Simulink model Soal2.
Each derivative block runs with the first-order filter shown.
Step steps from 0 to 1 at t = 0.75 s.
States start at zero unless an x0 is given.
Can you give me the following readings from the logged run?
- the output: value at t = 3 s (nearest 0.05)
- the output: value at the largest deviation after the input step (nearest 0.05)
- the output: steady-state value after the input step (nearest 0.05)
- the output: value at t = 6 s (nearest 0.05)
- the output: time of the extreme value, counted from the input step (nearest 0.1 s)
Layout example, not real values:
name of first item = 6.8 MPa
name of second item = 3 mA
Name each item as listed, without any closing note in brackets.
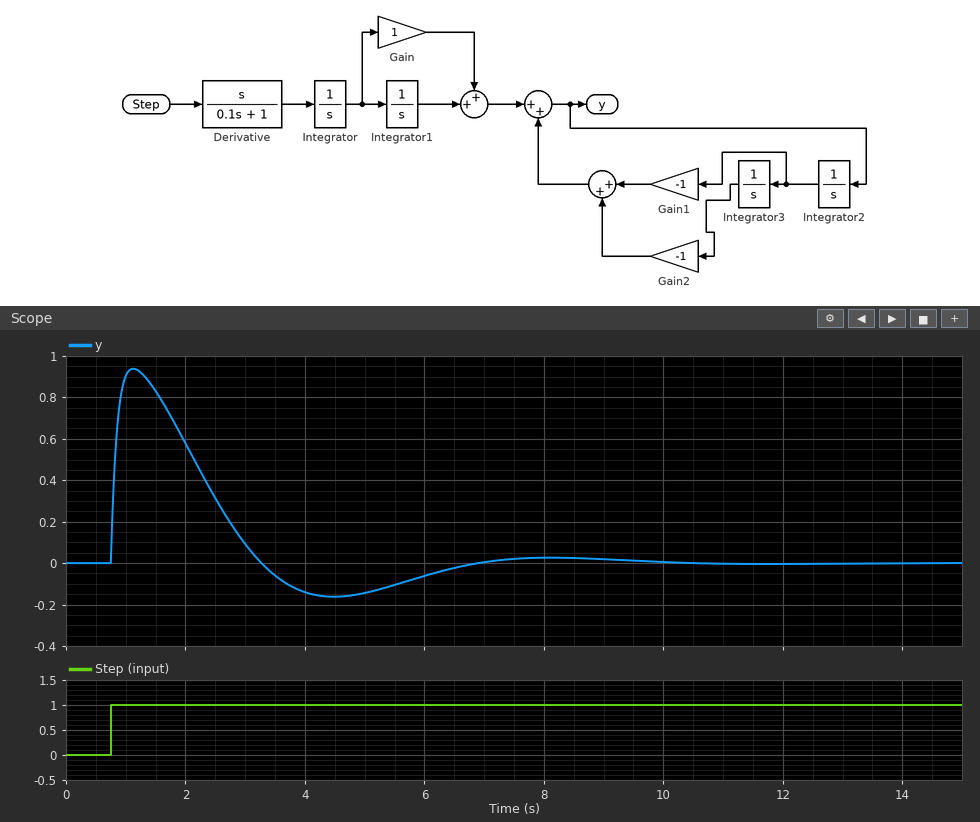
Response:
the output: value at t = 3 s = 0.10
the output: value at the largest deviation after the input step = 0.95
the output: steady-state value after the input step = 0.00
the output: value at t = 6 s = -0.05
the output: time of the extreme value, counted from the input step = 0.4 s
